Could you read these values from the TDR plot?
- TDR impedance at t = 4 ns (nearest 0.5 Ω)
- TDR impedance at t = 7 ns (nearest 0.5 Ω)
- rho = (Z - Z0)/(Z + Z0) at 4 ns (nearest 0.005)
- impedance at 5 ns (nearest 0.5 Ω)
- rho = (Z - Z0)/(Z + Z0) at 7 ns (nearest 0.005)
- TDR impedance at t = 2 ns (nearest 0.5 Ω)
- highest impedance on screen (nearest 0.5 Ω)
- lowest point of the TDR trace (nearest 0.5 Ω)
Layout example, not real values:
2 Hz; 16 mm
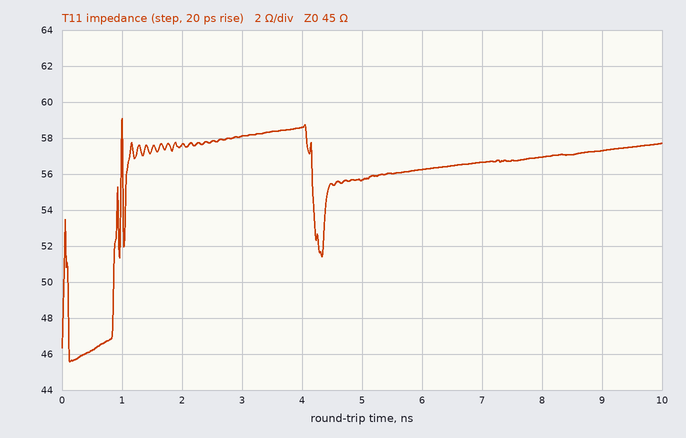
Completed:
58.5 Ω; 56.5 Ω; +0.130; 55.5 Ω; +0.115; 57.5 Ω; 59.0 Ω; 45.5 Ω
